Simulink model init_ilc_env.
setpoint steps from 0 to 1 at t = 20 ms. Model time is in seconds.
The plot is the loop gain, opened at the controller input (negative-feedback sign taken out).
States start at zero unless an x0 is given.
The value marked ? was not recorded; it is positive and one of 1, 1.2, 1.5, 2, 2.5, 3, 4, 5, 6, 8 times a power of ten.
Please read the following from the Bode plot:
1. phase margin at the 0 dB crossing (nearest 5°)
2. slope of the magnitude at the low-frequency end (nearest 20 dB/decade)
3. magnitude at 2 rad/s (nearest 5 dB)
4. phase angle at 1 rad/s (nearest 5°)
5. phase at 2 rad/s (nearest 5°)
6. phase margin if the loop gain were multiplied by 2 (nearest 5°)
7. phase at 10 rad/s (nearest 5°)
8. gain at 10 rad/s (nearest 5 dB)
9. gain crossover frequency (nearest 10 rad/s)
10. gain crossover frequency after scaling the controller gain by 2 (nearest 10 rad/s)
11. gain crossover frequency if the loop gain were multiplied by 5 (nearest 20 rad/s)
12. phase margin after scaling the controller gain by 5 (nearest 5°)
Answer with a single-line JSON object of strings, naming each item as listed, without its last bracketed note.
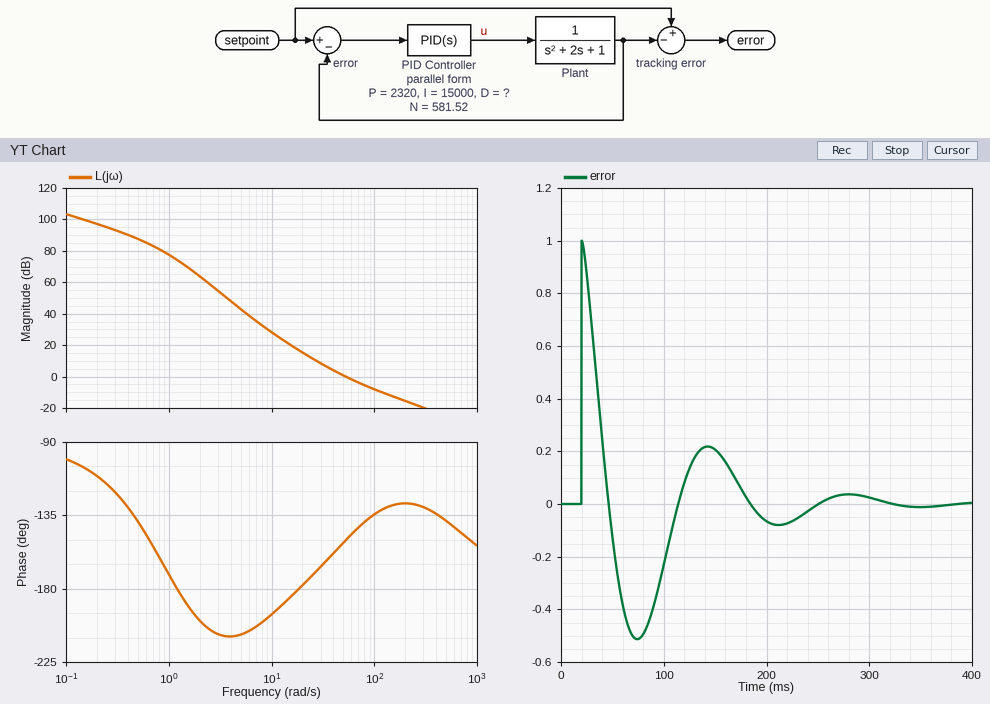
{"phase margin at the 0 dB crossing": "30°", "slope of the magnitude at the low-frequency end": "-20 dB/decade", "magnitude at 2 rad/s": "65 dB", "phase angle at 1 rad/s": "-170°", "phase at 2 rad/s": "-200°", "phase margin if the loop gain were multiplied by 2": "40°", "phase at 10 rad/s": "-195°", "gain at 10 rad/s": "30 dB", "gain crossover frequency": "50 rad/s", "gain crossover frequency after scaling the controller gain by 2": "80 rad/s", "gain crossover frequency if the loop gain were multiplied by 5": "180 rad/s", "phase margin after scaling the controller gain by 5": "50°"}
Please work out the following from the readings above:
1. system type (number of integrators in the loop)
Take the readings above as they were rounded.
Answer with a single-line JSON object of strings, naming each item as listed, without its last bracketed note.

{"system type": "1"}
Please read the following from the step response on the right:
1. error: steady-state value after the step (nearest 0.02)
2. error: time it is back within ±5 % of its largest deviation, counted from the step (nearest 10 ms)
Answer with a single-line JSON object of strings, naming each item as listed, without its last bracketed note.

{"error: steady-state value after the step": "0.00", "error: time it is back within ±5 % of its largest deviation, counted from the step": "210 ms"}
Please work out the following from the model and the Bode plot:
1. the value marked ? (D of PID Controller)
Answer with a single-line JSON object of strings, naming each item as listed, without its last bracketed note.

{"the value marked ?": "30"}
